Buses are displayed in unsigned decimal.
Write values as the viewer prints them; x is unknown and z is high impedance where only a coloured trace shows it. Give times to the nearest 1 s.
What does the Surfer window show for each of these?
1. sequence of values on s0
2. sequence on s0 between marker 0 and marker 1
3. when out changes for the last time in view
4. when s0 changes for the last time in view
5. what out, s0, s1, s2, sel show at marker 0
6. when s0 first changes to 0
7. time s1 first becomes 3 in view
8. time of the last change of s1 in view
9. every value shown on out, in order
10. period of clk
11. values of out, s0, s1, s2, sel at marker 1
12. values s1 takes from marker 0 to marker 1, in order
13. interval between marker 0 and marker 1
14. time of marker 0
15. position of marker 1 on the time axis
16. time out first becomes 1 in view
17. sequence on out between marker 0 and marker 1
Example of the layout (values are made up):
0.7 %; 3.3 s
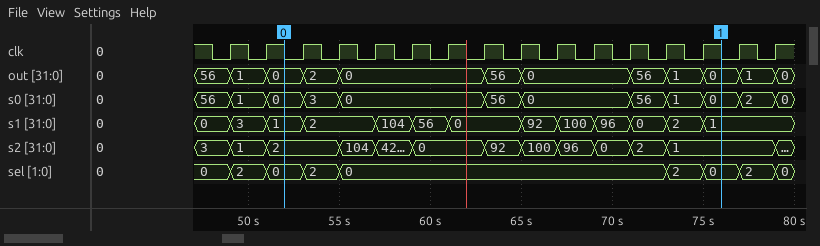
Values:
56, 1, 0, 3, 0, 56, 0, 56, 1, 0, 2, 0; 0, 3, 0, 56, 0, 56, 1, 0; 79 s; 79 s; out=0, s0=0, s1=1, s2=2, sel=0; 51 s; 49 s; 75 s; 56, 1, 0, 2, 0, 56, 0, 56, 1, 0, 1, 0; 2 s; out=0, s0=0, s1=1, s2=1, sel=0; 1, 2, 104, 56, 0, 92, 100, 96, 0, 2, 1; 24 s; 52 s; 76 s; 49 s; 0, 2, 0, 56, 0, 56, 1, 0
